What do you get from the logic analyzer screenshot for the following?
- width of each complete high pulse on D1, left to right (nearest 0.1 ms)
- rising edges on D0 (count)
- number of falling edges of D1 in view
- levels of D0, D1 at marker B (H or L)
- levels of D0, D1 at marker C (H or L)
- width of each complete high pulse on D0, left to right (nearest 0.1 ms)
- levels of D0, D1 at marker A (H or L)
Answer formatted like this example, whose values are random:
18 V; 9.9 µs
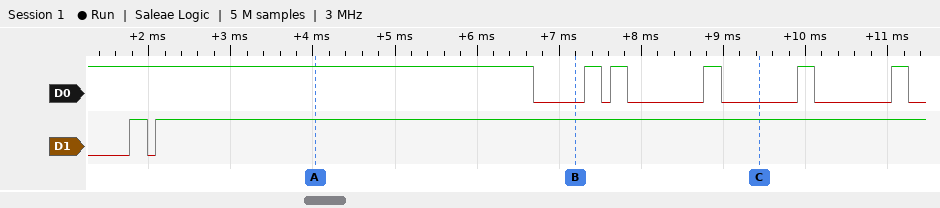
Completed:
0.2 ms; 5; 1; D0=L, D1=H; D0=L, D1=H; 0.2 ms, 0.2 ms, 0.2 ms, 0.2 ms, 0.2 ms; D0=H, D1=H
